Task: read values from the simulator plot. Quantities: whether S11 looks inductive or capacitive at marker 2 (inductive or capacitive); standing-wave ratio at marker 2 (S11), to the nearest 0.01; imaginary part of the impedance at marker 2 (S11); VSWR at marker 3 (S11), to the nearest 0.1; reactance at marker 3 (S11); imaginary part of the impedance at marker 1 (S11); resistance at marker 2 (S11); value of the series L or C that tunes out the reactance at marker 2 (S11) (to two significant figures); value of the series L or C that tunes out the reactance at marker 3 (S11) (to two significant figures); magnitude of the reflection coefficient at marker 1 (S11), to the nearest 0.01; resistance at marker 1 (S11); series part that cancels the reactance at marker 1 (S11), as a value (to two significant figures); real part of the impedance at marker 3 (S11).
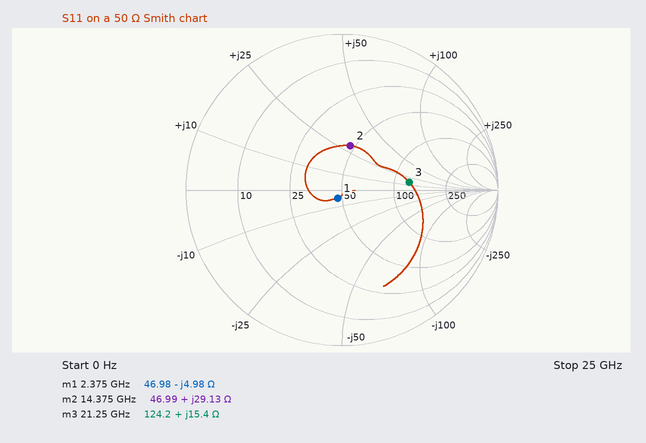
inductive
1.81
+29.13 Ω
2.5
+15.4 Ω
-4.98 Ω
46.99 Ω
380 fF
490 fF
0.06
46.98 Ω
330 pH
124.2 Ω
